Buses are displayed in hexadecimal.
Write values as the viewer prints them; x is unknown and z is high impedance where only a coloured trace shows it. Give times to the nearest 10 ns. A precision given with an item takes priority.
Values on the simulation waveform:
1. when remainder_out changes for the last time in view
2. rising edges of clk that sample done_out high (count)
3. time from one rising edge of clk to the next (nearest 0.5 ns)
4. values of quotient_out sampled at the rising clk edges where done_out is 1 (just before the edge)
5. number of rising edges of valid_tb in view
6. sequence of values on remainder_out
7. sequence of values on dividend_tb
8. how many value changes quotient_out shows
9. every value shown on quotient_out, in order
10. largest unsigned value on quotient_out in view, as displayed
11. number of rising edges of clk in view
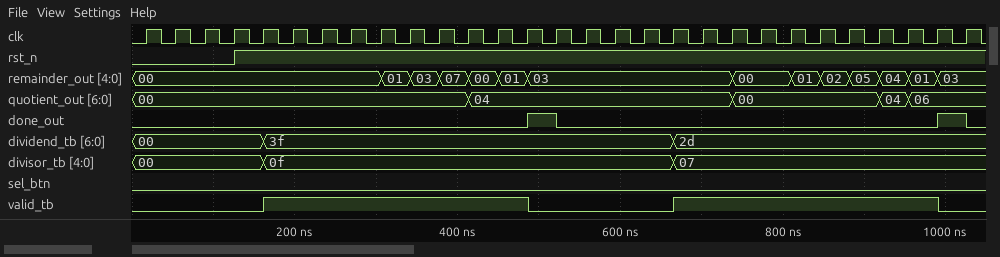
990 ns
2
36 ns
04, 06
2
00, 01, 03, 07, 00, 01, 03, 00, 01, 02, 05, 04, 01, 03
00, 3f, 2d
4
00, 04, 00, 04, 06
06
29
